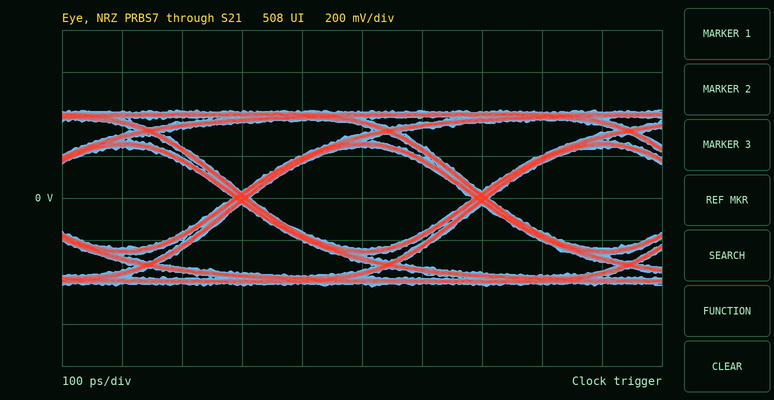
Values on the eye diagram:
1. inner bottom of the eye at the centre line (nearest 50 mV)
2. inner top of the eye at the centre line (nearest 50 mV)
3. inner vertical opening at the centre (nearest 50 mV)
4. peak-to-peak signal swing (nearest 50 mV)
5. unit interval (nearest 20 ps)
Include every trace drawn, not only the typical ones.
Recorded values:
-250 mV
250 mV
500 mV
850 mV
400 ps
